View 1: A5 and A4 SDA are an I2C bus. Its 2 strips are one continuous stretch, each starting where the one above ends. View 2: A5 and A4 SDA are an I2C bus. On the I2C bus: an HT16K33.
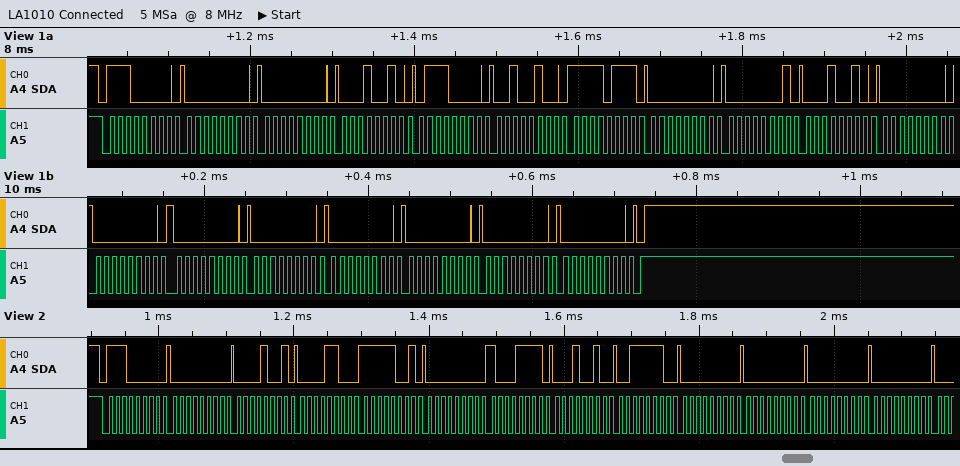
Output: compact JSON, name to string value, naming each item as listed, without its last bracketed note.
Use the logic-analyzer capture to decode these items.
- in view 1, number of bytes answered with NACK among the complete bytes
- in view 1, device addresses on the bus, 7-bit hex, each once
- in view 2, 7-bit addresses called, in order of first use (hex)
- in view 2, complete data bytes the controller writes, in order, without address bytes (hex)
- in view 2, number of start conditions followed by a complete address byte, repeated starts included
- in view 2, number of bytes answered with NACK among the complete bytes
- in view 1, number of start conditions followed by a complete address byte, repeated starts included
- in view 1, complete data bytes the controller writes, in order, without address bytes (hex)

{"in view 1, number of bytes answered with NACK among the complete bytes": "0", "in view 1, device addresses on the bus, 7-bit hex, each once": "0x70", "in view 2, 7-bit addresses called, in order of first use": "0x70", "in view 2, complete data bytes the controller writes, in order, without address bytes": "00 09 0C F9 00 8F 12 3E 00 00 00 00", "in view 2, number of start conditions followed by a complete address byte, repeated starts included": "1", "in view 2, number of bytes answered with NACK among the complete bytes": "0", "in view 1, number of start conditions followed by a complete address byte, repeated starts included": "1", "in view 1, complete data bytes the controller writes, in order, without address bytes": "00 00 12 70 24 F7 00 01 12 00 00 00 00 00 00 00 00"}
